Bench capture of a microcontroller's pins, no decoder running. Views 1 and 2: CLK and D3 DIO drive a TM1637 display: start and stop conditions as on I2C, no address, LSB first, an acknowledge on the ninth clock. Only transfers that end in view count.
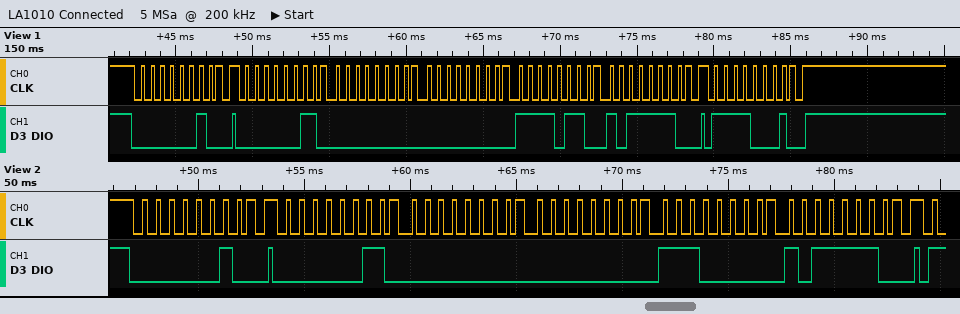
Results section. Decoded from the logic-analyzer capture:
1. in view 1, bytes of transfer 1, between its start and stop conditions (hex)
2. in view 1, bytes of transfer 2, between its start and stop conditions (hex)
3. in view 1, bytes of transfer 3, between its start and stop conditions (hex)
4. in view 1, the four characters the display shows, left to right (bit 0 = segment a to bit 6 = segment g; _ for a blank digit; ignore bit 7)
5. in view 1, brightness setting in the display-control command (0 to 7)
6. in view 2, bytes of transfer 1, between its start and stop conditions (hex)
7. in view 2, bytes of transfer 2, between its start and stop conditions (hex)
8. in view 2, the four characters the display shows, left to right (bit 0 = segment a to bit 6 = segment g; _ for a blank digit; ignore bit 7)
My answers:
40
C0 00 00 6F 7D
8F
__96
7
40
C0 00 00 07 7D
__76
